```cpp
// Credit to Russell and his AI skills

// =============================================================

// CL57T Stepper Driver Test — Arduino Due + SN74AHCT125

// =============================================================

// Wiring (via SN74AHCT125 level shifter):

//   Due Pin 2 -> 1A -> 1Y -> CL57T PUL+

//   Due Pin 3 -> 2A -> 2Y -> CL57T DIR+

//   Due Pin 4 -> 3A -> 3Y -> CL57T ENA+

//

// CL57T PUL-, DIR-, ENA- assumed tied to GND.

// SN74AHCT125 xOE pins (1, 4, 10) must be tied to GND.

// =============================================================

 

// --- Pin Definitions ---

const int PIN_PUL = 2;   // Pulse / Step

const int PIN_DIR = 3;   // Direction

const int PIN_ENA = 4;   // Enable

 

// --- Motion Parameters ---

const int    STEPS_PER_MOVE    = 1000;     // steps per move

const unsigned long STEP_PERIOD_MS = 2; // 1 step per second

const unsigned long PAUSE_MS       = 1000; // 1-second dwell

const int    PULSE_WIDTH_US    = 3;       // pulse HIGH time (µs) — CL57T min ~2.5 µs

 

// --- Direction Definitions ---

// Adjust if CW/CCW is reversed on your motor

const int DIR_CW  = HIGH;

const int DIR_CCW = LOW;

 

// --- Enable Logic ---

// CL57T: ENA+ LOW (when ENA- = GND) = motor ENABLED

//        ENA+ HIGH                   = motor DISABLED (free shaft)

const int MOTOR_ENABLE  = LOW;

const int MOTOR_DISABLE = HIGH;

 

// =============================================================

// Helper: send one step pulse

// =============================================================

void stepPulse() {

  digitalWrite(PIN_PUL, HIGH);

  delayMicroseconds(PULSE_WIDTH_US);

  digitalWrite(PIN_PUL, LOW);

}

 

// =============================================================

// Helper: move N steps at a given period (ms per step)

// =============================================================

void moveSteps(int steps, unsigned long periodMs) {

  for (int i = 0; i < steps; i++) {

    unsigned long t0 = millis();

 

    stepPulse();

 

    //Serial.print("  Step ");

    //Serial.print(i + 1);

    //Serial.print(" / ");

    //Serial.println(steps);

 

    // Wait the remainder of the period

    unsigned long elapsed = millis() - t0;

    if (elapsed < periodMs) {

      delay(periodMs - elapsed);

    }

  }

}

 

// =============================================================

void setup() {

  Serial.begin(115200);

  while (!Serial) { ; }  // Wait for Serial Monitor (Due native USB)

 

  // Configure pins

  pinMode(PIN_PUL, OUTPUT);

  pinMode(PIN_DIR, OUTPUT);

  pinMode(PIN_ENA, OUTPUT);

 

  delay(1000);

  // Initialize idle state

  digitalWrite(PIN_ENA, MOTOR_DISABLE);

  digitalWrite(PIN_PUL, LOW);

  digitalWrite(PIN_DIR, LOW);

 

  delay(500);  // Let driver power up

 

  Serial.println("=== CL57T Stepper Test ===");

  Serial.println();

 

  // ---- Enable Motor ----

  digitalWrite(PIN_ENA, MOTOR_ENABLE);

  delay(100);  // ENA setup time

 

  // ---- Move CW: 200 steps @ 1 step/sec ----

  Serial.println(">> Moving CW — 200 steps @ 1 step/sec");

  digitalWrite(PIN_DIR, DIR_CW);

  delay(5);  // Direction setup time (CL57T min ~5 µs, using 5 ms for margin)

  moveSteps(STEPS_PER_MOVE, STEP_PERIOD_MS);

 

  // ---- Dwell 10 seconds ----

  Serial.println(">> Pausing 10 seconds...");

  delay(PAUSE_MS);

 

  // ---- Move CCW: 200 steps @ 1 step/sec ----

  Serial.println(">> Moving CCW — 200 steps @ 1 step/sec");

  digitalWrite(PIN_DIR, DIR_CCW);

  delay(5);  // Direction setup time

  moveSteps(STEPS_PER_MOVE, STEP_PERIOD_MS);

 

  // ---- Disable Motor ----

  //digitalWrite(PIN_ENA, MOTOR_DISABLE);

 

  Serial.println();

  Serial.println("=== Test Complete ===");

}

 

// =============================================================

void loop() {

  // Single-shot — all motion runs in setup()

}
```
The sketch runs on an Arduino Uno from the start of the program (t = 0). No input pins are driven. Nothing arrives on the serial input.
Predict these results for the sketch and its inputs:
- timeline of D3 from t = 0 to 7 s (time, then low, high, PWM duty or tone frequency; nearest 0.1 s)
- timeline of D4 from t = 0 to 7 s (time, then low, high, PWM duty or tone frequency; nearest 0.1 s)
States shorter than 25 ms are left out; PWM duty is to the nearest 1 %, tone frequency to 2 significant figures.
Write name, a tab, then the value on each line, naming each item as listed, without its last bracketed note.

timeline of D3 from t = 0 to 7 s	0 s low; 1.6 s high; 4.6 s low
timeline of D4 from t = 0 to 7 s	0 s low; 1 s high; 1.5 s low
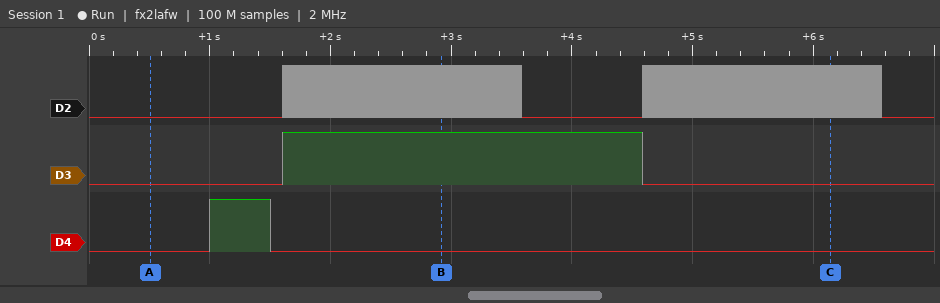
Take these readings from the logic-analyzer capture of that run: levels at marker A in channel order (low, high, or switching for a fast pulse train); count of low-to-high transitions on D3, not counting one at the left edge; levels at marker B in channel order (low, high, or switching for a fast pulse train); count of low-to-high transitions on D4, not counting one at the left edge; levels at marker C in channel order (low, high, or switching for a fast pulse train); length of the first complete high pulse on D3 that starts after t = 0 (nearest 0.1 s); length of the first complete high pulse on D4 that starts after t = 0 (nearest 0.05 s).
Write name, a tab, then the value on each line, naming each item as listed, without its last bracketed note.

levels at marker A in channel order	D2 low, D3 low, D4 low
count of low-to-high transitions on D3, not counting one at the left edge	1
levels at marker B in channel order	D2 switching, D3 high, D4 low
count of low-to-high transitions on D4, not counting one at the left edge	1
levels at marker C in channel order	D2 switching, D3 low, D4 low
length of the first complete high pulse on D3 that starts after t = 0	3.0 s
length of the first complete high pulse on D4 that starts after t = 0	0.50 s
